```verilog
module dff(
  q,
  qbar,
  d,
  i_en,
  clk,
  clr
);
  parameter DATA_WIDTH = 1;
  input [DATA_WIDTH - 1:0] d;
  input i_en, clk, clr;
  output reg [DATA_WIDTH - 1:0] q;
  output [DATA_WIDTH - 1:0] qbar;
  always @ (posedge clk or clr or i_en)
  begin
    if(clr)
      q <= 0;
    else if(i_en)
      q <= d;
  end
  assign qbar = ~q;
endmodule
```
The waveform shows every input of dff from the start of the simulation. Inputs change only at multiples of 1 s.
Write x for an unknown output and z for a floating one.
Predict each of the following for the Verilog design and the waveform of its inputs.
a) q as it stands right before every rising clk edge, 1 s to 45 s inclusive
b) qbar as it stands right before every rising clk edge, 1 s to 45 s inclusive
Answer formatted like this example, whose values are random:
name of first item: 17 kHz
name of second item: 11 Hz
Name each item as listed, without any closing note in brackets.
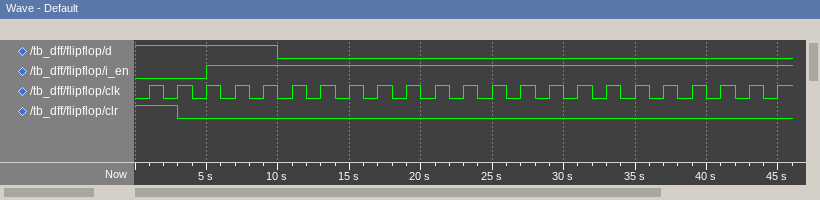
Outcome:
q as it stands right before every rising clk edge, 1 s to 45 s inclusive: 0 0 0 1 1 1 0 0 0 0 0 0 0 0 0 0 0 0 0 0 0 0 0
qbar as it stands right before every rising clk edge, 1 s to 45 s inclusive: 1 1 1 0 0 0 1 1 1 1 1 1 1 1 1 1 1 1 1 1 1 1 1
